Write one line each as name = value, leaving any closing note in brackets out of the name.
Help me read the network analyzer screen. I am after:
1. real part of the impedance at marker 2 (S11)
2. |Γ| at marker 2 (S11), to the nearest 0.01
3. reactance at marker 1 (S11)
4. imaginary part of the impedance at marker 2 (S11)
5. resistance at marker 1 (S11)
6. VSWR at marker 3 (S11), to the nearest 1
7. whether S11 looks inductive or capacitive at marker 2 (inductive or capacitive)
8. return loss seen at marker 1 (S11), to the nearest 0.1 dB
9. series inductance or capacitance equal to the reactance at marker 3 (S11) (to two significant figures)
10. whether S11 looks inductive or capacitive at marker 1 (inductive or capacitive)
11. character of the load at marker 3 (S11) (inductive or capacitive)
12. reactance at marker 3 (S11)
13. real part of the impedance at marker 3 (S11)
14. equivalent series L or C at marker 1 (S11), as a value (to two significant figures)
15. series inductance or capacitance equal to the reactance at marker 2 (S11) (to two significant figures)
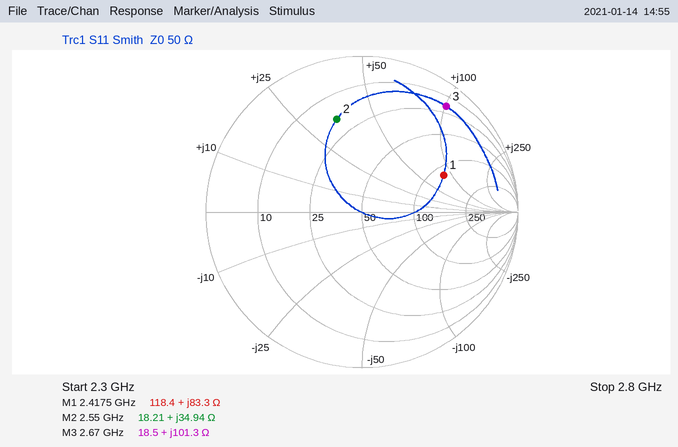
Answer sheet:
real part of the impedance at marker 2 = 18.21 Ω
|Γ| at marker 2 (S11), to the nearest 0.01 = 0.62
reactance at marker 1 = +83.3 Ω
imaginary part of the impedance at marker 2 = +34.94 Ω
resistance at marker 1 = 118.4 Ω
VSWR at marker 3 (S11), to the nearest 1 = 14
whether S11 looks inductive or capacitive at marker 2 = inductive
return loss seen at marker 1 (S11), to the nearest 0.1 dB = 4.8 dB
series inductance or capacitance equal to the reactance at marker 3 (S11) = 6.0 nH
whether S11 looks inductive or capacitive at marker 1 = inductive
character of the load at marker 3 (S11) = inductive
reactance at marker 3 = +101.3 Ω
real part of the impedance at marker 3 = 18.5 Ω
equivalent series L or C at marker 1 (S11), as a value = 5.5 nH
series inductance or capacitance equal to the reactance at marker 2 (S11) = 2.2 nH
